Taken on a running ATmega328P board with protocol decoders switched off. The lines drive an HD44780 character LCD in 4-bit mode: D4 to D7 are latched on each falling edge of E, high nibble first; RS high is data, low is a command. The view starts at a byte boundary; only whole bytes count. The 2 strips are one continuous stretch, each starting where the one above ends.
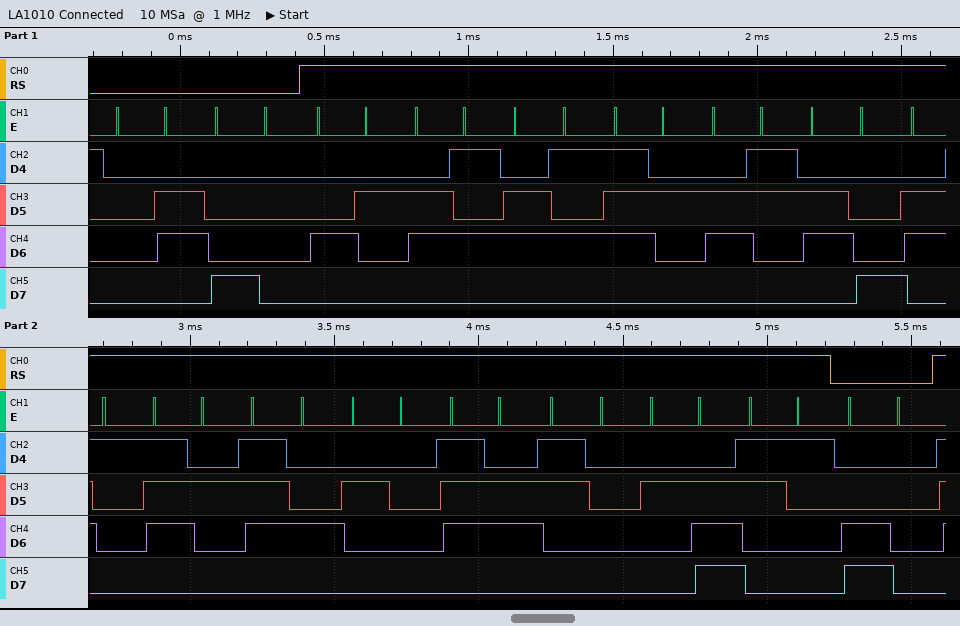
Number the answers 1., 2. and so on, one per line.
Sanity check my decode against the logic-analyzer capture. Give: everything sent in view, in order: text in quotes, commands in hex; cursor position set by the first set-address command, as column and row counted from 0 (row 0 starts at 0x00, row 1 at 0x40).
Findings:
1. 0x06 0x80 "Beerchart v0.1" 0xC0
2. column 0, row 0
